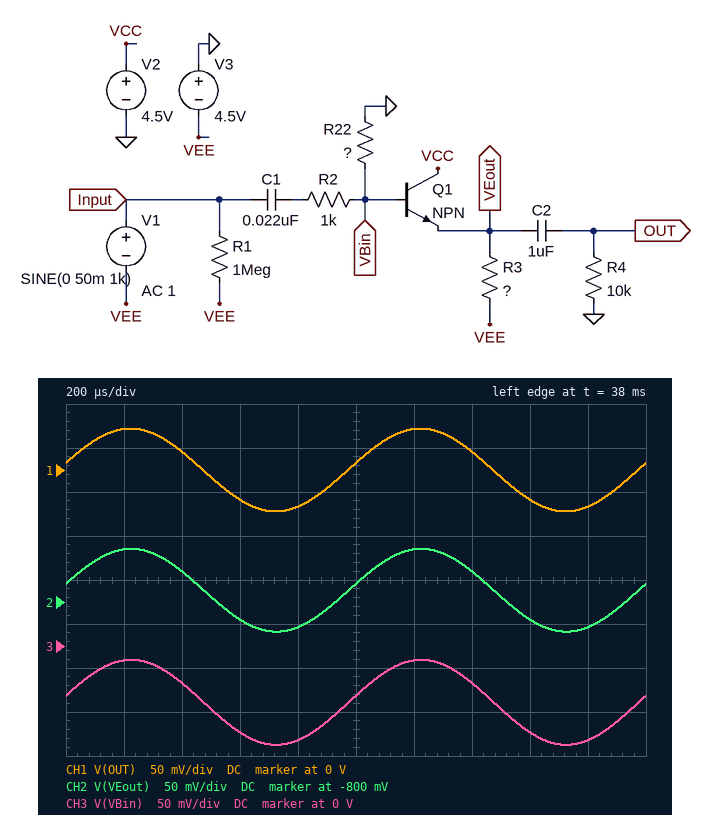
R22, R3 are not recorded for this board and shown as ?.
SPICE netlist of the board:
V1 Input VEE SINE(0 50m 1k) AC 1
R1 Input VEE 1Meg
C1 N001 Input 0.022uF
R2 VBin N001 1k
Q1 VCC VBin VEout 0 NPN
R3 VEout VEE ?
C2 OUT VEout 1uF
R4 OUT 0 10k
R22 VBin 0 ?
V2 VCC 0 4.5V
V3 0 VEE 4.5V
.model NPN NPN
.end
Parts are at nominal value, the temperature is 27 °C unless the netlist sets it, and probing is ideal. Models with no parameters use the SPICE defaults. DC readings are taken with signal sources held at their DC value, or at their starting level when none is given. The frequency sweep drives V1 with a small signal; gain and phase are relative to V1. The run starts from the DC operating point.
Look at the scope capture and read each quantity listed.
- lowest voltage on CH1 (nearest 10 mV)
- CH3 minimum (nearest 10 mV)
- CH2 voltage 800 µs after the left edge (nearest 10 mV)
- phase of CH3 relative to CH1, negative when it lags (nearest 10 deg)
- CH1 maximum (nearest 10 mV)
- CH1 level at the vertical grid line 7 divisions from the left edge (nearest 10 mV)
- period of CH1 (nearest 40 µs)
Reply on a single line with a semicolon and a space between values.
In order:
-50 mV; -110 mV; -830 mV; 0 deg; 50 mV; 20 mV; 1.00 ms
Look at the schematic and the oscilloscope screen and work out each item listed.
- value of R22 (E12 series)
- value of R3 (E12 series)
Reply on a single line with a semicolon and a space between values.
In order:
47 kΩ; 27 kΩ
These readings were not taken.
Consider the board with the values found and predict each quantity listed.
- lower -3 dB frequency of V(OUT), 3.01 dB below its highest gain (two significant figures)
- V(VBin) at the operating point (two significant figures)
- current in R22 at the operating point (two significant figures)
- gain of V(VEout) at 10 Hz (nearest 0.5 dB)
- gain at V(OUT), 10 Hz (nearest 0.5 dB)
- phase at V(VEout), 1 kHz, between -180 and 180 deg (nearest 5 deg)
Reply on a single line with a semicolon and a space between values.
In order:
160 Hz; -64 mV; 1.4 µA; -24.0 dB; -29.5 dB; 10 deg
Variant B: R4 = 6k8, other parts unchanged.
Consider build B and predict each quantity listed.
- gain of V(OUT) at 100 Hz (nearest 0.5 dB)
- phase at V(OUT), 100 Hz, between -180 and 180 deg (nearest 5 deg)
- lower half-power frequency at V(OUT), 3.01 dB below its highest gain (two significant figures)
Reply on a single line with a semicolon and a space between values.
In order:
-6.5 dB; 70 deg; 170 Hz
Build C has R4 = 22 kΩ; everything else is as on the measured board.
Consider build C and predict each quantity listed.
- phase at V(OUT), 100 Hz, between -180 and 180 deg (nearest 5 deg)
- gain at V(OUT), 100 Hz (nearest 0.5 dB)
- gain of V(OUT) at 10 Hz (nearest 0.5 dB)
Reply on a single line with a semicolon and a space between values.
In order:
60 deg; -5.5 dB; -26.0 dB
